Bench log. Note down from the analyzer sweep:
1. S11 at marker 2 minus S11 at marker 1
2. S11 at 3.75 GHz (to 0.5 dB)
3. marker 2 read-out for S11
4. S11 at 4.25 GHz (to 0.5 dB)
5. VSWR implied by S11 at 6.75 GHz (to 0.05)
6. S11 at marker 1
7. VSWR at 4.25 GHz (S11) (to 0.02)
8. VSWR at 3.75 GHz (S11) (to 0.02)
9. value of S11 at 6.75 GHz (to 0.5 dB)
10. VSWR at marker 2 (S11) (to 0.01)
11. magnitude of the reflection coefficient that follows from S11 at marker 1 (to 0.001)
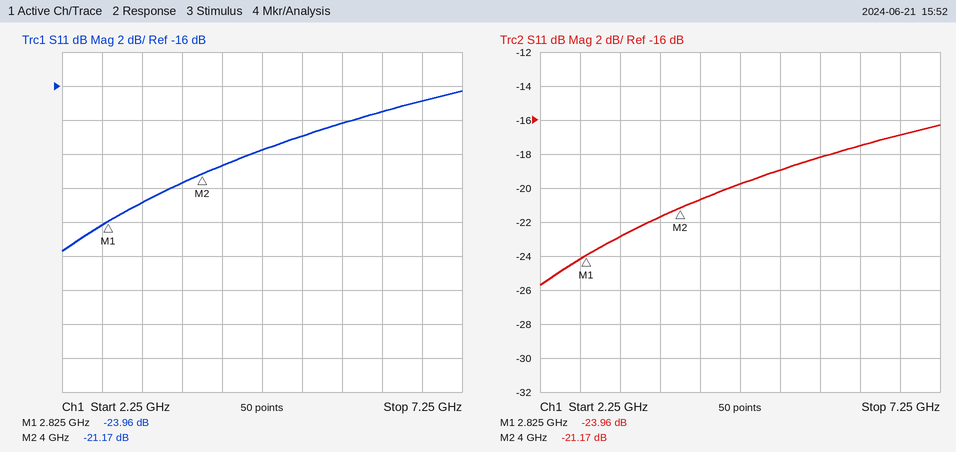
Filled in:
2.79 dB
-21.5 dB
-21.17 dB
-20.5 dB
1.35
-23.96 dB
1.20
1.18
-17.0 dB
1.19
0.063
